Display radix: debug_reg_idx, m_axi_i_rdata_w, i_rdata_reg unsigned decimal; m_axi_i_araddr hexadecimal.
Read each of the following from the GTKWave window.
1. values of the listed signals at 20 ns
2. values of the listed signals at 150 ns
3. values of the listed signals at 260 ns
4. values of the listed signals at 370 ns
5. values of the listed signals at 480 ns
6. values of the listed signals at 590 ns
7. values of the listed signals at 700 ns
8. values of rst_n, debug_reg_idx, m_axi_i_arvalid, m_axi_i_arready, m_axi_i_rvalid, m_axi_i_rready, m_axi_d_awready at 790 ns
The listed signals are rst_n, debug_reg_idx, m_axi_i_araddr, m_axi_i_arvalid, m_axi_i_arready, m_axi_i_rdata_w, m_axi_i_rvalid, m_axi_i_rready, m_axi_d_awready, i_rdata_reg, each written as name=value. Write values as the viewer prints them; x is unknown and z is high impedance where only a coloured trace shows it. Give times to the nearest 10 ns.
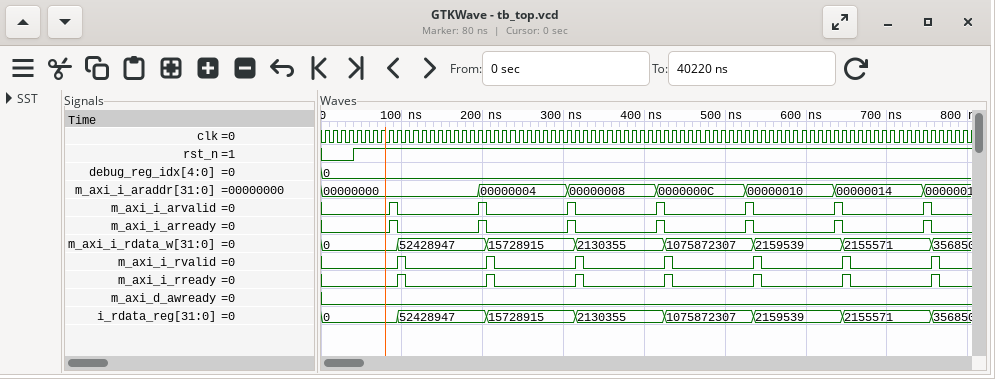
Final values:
rst_n=0, debug_reg_idx=0, m_axi_i_araddr=00000000, m_axi_i_arvalid=0, m_axi_i_arready=0, m_axi_i_rdata_w=0, m_axi_i_rvalid=0, m_axi_i_rready=0, m_axi_d_awready=0, i_rdata_reg=0
rst_n=1, debug_reg_idx=0, m_axi_i_araddr=00000000, m_axi_i_arvalid=0, m_axi_i_arready=0, m_axi_i_rdata_w=52428947, m_axi_i_rvalid=0, m_axi_i_rready=0, m_axi_d_awready=0, i_rdata_reg=52428947
rst_n=1, debug_reg_idx=0, m_axi_i_araddr=00000004, m_axi_i_arvalid=0, m_axi_i_arready=0, m_axi_i_rdata_w=15728915, m_axi_i_rvalid=0, m_axi_i_rready=0, m_axi_d_awready=0, i_rdata_reg=15728915
rst_n=1, debug_reg_idx=0, m_axi_i_araddr=00000008, m_axi_i_arvalid=0, m_axi_i_arready=0, m_axi_i_rdata_w=2130355, m_axi_i_rvalid=0, m_axi_i_rready=0, m_axi_d_awready=0, i_rdata_reg=2130355
rst_n=1, debug_reg_idx=0, m_axi_i_araddr=0000000C, m_axi_i_arvalid=0, m_axi_i_arready=0, m_axi_i_rdata_w=1075872307, m_axi_i_rvalid=0, m_axi_i_rready=0, m_axi_d_awready=0, i_rdata_reg=1075872307
rst_n=1, debug_reg_idx=0, m_axi_i_araddr=00000010, m_axi_i_arvalid=0, m_axi_i_arready=0, m_axi_i_rdata_w=2159539, m_axi_i_rvalid=0, m_axi_i_rready=0, m_axi_d_awready=0, i_rdata_reg=2159539
rst_n=1, debug_reg_idx=0, m_axi_i_araddr=00000014, m_axi_i_arvalid=0, m_axi_i_arready=0, m_axi_i_rdata_w=2155571, m_axi_i_rvalid=0, m_axi_i_rready=0, m_axi_d_awready=0, i_rdata_reg=2155571
rst_n=1, debug_reg_idx=0, m_axi_i_arvalid=0, m_axi_i_arready=0, m_axi_i_rvalid=0, m_axi_i_rready=0, m_axi_d_awready=0
